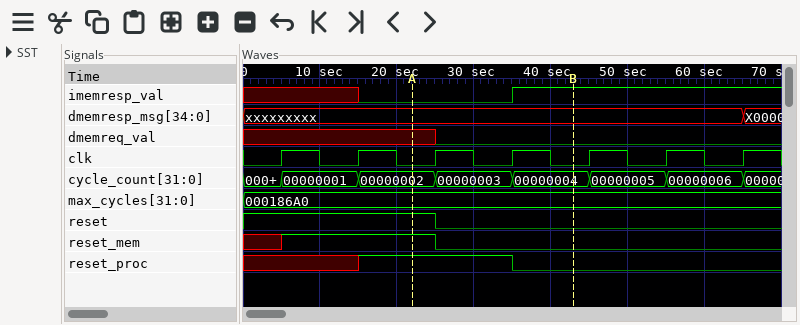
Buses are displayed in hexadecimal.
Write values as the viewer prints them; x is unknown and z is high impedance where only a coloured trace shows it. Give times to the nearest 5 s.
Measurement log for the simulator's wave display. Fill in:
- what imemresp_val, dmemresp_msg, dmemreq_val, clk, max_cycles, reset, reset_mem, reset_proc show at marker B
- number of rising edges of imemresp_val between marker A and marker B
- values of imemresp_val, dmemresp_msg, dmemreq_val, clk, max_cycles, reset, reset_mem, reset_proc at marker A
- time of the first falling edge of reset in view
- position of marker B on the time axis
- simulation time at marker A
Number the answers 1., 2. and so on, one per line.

1. imemresp_val=1, dmemresp_msg=xxxxxxxxx, dmemreq_val=0, clk=0, max_cycles=000186A0, reset=0, reset_mem=0, reset_proc=0
2. 1
3. imemresp_val=0, dmemresp_msg=xxxxxxxxx, dmemreq_val=x, clk=0, max_cycles=000186A0, reset=1, reset_mem=1, reset_proc=1
4. 25 s
5. 45 s
6. 20 s
